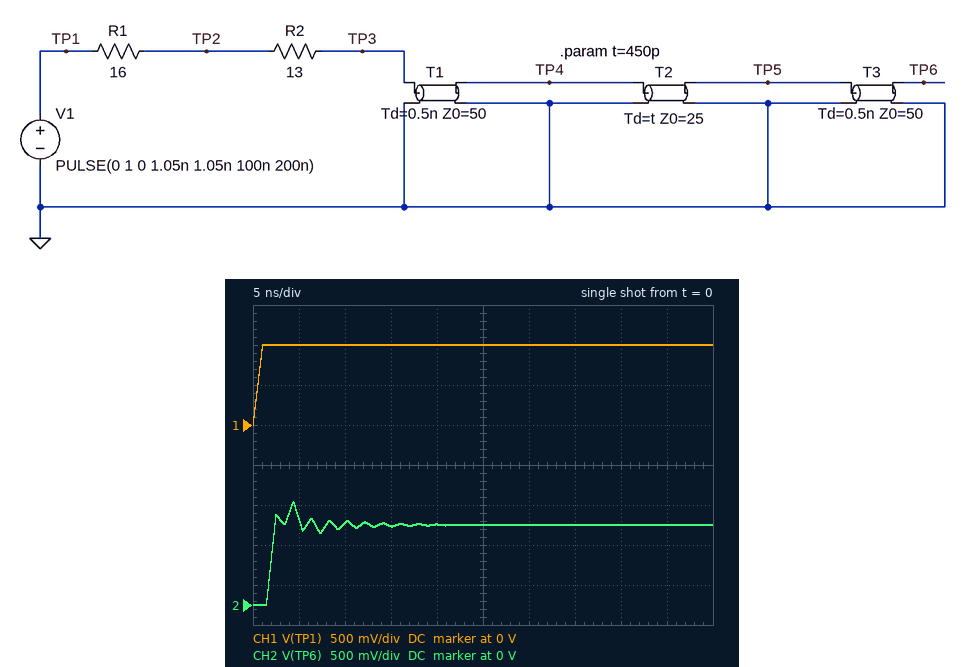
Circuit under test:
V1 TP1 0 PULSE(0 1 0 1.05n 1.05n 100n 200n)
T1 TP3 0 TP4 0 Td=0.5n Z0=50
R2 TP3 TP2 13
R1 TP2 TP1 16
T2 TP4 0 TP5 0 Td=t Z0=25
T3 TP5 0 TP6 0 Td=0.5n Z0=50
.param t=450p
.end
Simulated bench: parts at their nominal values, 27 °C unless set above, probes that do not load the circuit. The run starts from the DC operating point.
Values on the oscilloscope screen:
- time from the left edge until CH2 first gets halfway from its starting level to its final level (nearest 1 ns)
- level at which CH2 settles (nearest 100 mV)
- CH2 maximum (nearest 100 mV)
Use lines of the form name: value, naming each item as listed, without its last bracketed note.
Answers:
time from the left edge until CH2 first gets halfway from its starting level to its final level: 2 ns
level at which CH2 settles: 1.0 V
CH2 maximum: 1.3 V
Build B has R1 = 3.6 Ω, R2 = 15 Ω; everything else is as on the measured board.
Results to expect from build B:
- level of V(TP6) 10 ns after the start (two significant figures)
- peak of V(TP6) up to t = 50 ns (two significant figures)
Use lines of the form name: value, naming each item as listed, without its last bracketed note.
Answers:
level of V(TP6) 10 ns after the start: 1.1 V
peak of V(TP6) up to t = 50 ns: 1.5 V
